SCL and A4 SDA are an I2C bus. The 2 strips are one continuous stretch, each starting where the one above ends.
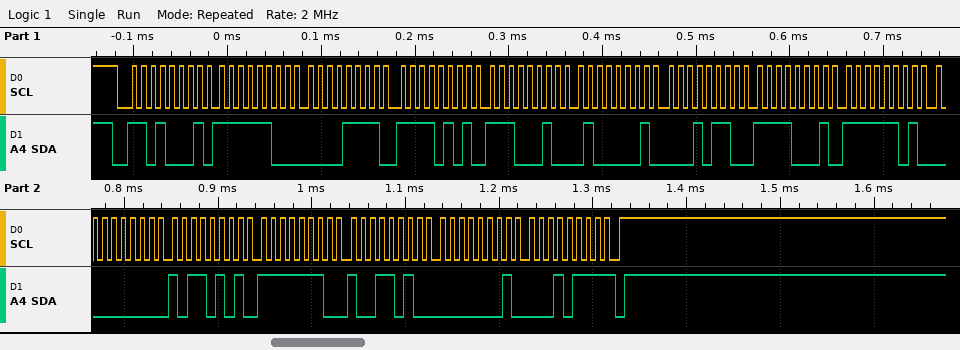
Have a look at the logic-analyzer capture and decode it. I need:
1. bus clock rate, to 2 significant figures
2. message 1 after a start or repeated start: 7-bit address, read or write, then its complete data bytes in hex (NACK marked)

100 kHz
0x68 read: FC 0F F5 E2 41 16 F1 FD 00 B5 FE 9A 01 17 NACK
